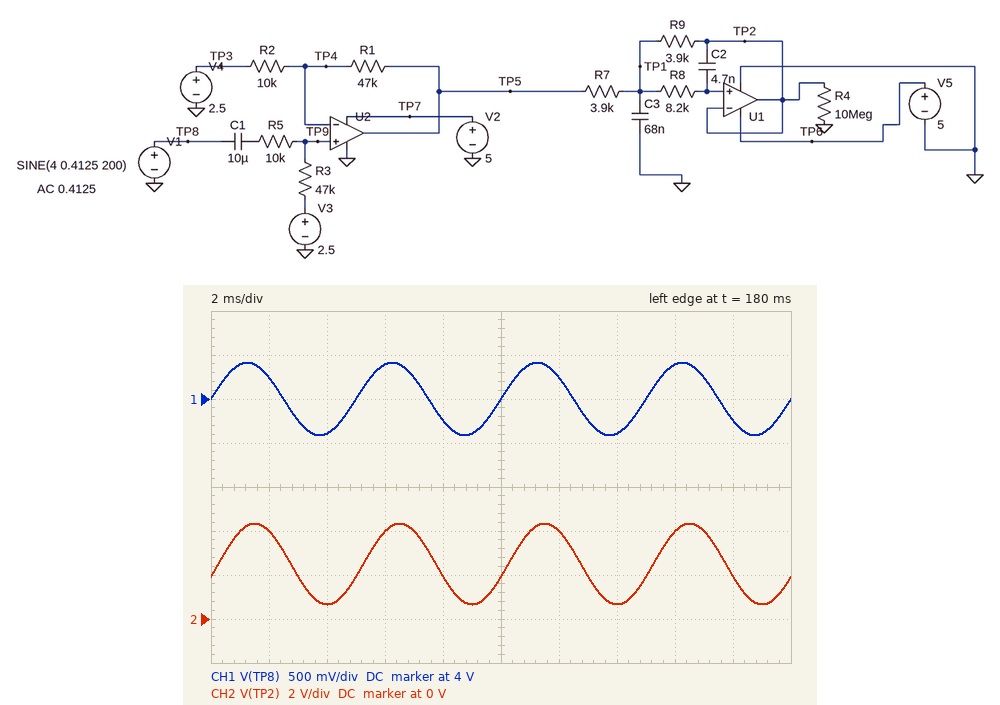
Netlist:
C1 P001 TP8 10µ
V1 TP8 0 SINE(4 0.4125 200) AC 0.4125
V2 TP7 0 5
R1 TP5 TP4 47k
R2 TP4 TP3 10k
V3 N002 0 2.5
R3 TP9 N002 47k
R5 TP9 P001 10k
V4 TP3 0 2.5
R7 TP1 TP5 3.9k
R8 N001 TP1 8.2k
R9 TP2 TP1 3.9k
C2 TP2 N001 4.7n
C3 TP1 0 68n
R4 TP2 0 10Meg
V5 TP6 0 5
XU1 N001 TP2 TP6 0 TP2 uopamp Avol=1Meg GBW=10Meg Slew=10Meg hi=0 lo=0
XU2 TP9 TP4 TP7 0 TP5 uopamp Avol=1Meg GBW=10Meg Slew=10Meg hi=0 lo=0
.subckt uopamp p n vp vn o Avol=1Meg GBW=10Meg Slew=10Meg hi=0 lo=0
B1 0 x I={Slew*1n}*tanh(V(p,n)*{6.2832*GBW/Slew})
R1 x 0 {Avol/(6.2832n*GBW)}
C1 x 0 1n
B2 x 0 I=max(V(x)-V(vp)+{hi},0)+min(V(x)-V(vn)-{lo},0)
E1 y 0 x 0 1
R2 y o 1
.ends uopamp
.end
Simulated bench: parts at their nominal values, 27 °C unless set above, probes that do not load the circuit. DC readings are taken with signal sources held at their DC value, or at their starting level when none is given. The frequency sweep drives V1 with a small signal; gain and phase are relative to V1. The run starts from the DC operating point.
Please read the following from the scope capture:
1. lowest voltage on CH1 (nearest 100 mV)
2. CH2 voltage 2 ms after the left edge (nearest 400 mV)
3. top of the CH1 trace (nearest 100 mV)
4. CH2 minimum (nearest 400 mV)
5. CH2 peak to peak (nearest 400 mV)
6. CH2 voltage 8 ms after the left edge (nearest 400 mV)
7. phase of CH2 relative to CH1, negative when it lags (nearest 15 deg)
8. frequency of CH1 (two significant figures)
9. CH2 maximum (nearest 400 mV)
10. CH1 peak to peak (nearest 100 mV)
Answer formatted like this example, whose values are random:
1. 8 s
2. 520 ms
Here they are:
1. 3.6 V
2. 4.0 V
3. 4.4 V
4. 800 mV
5. 3.6 V
6. 2.0 V
7. -15 deg
8. 200 Hz
9. 4.4 V
10. 800 mV
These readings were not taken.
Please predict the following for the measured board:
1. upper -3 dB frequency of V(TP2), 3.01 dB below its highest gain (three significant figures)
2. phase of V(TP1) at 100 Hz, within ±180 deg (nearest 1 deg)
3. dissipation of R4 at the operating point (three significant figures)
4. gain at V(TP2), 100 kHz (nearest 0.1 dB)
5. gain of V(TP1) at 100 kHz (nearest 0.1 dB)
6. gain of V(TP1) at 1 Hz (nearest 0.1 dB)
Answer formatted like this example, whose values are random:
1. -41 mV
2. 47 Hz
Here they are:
1. 601 Hz
2. -9 deg
3. 625 nW
4. -28.6 dB
5. -31.0 dB
6. 13.1 dB
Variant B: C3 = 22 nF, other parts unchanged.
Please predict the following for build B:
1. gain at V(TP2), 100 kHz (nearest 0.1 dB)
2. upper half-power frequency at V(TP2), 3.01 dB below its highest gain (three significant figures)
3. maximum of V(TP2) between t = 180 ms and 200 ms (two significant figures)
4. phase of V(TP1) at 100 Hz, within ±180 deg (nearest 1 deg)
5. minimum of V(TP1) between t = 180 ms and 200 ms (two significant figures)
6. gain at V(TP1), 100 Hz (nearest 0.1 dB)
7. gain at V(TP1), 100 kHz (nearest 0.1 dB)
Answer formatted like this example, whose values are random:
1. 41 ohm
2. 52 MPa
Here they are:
1. -18.8 dB
2. 1.86 kHz
3. 4.4 V
4. -3 deg
5. 570 mV
6. 13.4 dB
7. -21.2 dB
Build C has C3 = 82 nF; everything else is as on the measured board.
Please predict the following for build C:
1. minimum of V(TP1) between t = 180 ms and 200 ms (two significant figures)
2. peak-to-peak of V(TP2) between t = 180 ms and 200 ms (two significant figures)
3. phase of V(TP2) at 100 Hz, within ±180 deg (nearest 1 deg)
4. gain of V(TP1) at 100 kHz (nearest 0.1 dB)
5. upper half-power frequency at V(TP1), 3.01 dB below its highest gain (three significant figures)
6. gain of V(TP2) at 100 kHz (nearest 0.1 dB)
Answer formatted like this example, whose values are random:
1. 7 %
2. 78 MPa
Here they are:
1. 700 mV
2. 3.6 V
3. -11 deg
4. -32.6 dB
5. 498 Hz
6. -30.2 dB
